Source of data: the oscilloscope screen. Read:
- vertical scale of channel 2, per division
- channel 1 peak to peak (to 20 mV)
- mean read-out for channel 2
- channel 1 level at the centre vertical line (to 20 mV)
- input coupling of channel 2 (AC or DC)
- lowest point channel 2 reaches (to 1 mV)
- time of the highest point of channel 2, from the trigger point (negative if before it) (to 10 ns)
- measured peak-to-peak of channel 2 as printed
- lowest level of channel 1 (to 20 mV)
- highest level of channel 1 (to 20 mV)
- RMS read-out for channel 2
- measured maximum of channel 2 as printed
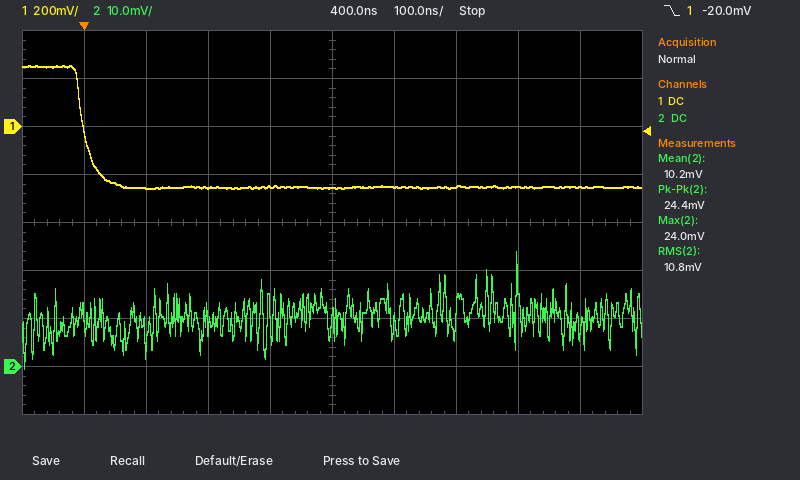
10 mV
520 mV
10.2 mV
-260 mV
DC
0 mV
+700 ns
24.4 mV
-260 mV
260 mV
10.8 mV
24.0 mV
